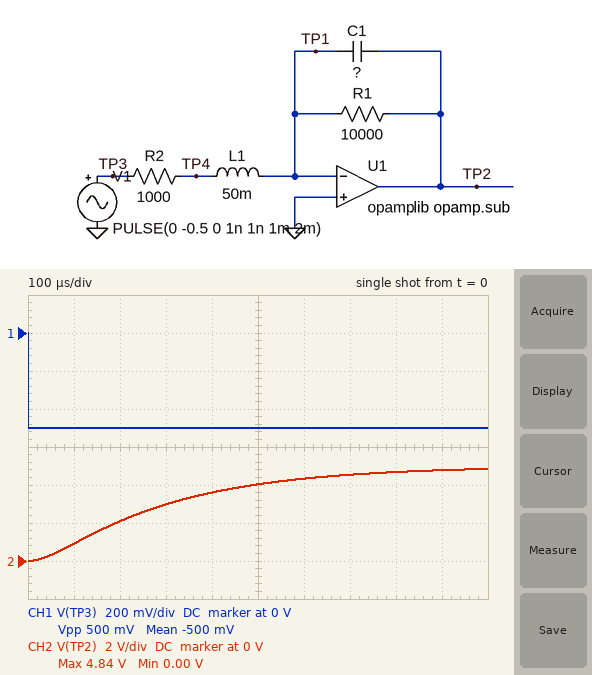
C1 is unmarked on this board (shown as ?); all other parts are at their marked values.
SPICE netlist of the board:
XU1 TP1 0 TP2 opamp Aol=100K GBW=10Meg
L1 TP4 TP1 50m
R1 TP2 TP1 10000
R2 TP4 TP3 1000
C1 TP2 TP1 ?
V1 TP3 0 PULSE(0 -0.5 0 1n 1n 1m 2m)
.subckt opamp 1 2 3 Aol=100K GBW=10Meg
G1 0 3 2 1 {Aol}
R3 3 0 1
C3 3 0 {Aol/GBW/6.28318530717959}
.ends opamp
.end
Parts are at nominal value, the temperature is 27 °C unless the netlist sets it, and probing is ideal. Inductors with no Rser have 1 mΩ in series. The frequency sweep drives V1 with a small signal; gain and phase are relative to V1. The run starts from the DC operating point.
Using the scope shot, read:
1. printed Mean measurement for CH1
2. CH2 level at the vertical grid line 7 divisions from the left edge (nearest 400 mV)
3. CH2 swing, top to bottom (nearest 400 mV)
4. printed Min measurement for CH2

-500 mV
4.4 V
4.8 V
0.00 V
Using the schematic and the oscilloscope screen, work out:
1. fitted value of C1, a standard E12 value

27 nF
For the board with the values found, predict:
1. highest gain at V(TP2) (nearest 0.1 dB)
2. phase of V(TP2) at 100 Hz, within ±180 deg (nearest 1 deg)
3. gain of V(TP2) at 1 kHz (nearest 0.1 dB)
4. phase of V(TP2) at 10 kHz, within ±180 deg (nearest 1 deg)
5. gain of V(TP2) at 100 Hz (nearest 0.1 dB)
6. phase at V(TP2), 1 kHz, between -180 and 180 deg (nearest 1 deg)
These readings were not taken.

20.0 dB
169 deg
13.7 dB
21 deg
19.9 dB
103 deg
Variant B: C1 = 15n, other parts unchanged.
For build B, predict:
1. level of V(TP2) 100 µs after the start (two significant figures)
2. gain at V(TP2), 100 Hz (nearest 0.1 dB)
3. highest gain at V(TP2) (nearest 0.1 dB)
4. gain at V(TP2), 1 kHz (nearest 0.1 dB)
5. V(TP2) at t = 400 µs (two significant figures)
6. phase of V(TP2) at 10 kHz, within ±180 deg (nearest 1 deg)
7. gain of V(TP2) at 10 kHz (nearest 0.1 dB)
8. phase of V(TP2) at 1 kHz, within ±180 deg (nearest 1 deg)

1.5 V
20.0 dB
20.0 dB
16.8 dB
4.5 V
24 deg
-9.9 dB
119 deg
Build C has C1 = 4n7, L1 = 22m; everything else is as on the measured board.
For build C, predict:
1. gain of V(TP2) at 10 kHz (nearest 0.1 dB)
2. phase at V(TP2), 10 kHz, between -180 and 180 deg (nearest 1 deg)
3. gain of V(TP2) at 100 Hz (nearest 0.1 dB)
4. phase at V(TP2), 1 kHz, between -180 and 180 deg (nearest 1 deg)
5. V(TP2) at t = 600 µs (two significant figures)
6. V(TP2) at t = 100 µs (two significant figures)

5.5 dB
55 deg
20.0 dB
156 deg
5.0 V
3.9 V
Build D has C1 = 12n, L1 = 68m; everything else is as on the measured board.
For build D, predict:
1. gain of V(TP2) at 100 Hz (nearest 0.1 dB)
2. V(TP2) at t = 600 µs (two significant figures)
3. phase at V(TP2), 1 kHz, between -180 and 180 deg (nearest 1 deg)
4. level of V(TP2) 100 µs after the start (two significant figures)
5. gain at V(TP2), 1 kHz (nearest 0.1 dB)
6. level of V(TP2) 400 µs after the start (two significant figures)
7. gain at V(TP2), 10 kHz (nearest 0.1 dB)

20.0 dB
4.9 V
120 deg
1.5 V
17.3 dB
4.6 V
-10.5 dB
